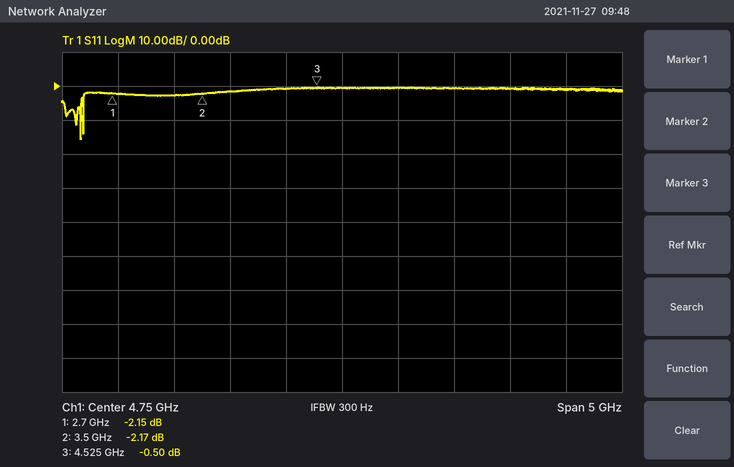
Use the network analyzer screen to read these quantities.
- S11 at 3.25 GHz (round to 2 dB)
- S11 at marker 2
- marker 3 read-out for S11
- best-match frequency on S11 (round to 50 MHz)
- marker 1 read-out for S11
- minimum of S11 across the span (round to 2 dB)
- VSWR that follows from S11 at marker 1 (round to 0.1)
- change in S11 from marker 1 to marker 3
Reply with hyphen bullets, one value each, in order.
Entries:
- -2 dB
- -2.17 dB
- -0.50 dB
- 2.40 GHz
- -2.15 dB
- -16 dB
- 8.1
- 1.65 dB
